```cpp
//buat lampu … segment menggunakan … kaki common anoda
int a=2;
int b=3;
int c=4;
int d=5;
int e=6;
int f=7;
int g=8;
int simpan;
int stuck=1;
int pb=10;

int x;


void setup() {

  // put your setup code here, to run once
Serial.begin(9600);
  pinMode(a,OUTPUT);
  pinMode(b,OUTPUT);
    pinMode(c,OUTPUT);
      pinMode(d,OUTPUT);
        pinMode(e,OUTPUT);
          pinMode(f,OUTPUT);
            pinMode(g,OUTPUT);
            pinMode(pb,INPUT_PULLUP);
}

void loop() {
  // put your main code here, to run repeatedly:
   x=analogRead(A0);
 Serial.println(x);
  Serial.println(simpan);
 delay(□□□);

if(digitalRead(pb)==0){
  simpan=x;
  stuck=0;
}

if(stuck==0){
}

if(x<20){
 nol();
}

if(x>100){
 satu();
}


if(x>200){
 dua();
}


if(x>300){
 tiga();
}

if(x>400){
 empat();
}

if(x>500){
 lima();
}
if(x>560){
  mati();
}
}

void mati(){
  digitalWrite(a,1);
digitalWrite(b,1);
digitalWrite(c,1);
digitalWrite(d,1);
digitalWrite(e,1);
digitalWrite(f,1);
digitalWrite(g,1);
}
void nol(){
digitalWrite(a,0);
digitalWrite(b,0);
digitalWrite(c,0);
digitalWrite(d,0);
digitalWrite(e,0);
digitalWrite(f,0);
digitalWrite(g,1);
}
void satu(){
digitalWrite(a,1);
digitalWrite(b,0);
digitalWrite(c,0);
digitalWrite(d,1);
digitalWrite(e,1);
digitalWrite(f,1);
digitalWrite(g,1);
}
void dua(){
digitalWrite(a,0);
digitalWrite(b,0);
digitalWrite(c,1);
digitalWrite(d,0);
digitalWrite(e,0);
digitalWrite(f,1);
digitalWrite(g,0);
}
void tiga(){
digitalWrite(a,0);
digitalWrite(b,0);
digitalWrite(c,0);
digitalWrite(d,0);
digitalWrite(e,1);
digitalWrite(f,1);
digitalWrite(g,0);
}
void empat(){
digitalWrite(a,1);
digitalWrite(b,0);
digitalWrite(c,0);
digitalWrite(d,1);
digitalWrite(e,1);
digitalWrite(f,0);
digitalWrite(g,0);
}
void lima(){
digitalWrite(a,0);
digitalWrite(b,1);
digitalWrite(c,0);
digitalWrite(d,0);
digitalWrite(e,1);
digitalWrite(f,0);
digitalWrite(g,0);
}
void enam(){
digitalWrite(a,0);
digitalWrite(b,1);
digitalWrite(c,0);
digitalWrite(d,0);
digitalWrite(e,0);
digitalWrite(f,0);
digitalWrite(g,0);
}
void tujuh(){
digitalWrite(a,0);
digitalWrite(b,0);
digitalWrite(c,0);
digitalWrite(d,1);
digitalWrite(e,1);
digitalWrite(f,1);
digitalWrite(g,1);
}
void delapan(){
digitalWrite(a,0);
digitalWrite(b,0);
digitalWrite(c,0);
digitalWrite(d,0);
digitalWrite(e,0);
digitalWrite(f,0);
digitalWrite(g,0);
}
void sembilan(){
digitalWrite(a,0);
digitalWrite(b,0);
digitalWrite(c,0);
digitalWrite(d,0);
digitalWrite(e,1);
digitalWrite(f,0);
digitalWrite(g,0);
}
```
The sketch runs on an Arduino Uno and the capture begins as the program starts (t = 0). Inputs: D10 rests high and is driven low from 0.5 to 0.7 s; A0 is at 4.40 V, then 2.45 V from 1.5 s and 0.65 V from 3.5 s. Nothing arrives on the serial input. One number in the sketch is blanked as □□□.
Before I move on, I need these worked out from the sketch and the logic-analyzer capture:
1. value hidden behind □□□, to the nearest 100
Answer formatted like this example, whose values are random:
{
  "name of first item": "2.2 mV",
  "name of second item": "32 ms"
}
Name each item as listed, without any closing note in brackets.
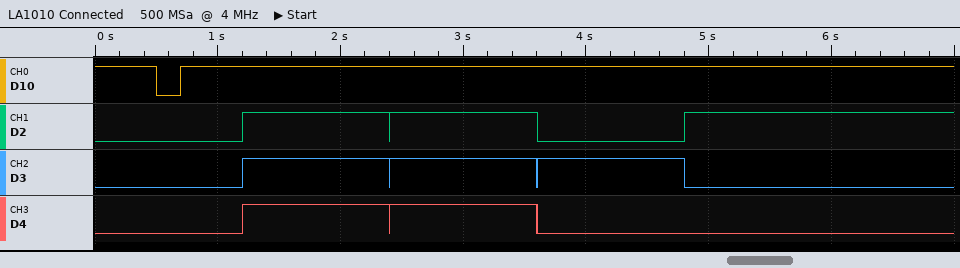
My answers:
{
  "value hidden behind □□□, to the nearest 100": "1200"
}
